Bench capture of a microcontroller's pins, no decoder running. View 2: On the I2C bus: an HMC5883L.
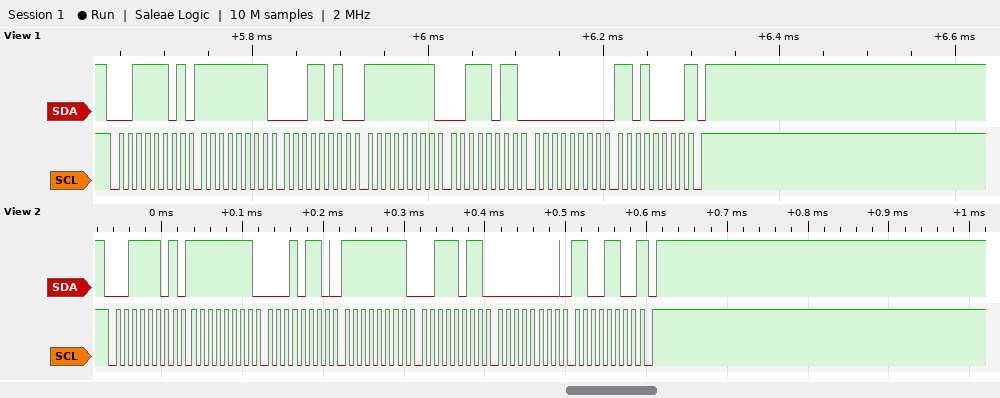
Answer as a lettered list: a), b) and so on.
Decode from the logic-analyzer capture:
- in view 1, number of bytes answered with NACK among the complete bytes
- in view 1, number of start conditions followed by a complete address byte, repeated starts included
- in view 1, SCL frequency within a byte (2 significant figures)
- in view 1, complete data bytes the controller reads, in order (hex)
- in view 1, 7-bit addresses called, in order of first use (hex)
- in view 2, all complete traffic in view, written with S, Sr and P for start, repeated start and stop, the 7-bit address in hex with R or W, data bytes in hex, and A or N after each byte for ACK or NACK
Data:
a) 1
b) 1
c) 100 kHz
d) FF 1A FF 3B 00 D0
e) 0x1E
f) S 1ER A FF A 16 A FF A 3B A 00 A CC N P
